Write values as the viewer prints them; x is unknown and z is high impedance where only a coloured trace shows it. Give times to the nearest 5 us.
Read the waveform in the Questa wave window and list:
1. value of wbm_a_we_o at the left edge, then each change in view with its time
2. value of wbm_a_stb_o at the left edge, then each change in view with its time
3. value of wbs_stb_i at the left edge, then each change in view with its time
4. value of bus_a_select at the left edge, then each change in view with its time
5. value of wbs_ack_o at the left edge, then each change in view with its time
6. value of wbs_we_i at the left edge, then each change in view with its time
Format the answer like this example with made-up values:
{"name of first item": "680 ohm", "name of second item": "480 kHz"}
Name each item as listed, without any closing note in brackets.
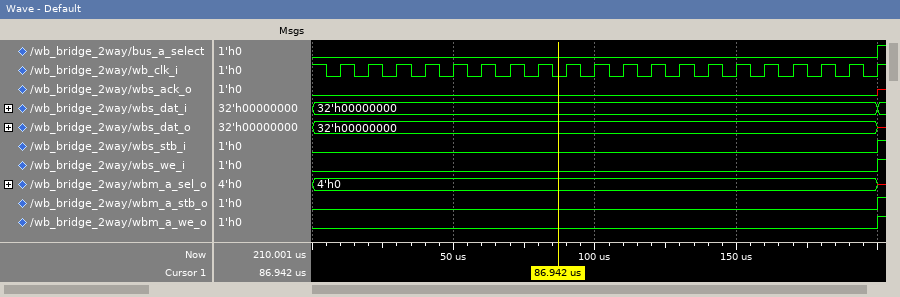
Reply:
{"value of wbm_a_we_o at the left edge, then each change in view with its time": "0, 1 at 200 us", "value of wbm_a_stb_o at the left edge, then each change in view with its time": "0, 1 at 200 us", "value of wbs_stb_i at the left edge, then each change in view with its time": "0, 1 at 200 us", "value of bus_a_select at the left edge, then each change in view with its time": "0, 1 at 200 us", "value of wbs_ack_o at the left edge, then each change in view with its time": "0, x at 200 us", "value of wbs_we_i at the left edge, then each change in view with its time": "0, 1 at 200 us"}
